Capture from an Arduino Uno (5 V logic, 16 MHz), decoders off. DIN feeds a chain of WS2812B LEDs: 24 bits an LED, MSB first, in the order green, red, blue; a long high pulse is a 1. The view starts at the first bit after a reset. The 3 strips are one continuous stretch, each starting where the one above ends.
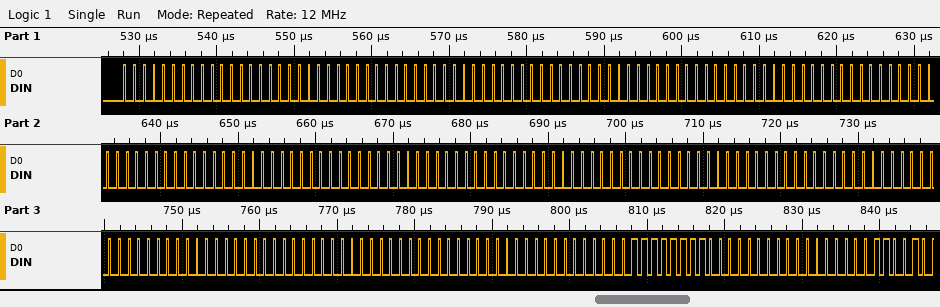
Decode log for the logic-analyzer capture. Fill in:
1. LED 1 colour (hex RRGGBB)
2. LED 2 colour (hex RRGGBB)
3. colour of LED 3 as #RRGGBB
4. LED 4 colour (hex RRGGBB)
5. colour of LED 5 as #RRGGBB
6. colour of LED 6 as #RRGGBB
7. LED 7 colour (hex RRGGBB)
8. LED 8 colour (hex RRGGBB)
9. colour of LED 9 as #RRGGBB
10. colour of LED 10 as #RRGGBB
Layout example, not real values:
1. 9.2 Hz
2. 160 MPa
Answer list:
1. #000000
2. #000000
3. #000000
4. #000000
5. #000000
6. #000000
7. #000000
8. #000000
9. #000000
10. #FF0000
